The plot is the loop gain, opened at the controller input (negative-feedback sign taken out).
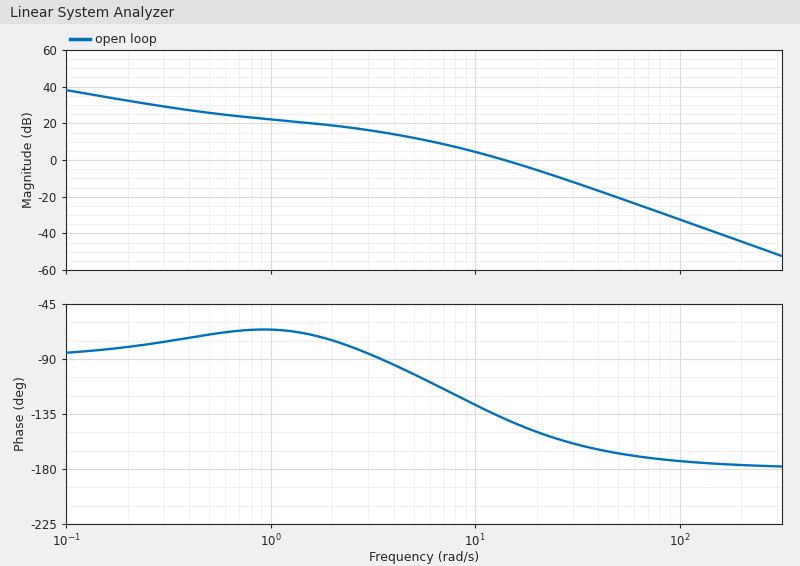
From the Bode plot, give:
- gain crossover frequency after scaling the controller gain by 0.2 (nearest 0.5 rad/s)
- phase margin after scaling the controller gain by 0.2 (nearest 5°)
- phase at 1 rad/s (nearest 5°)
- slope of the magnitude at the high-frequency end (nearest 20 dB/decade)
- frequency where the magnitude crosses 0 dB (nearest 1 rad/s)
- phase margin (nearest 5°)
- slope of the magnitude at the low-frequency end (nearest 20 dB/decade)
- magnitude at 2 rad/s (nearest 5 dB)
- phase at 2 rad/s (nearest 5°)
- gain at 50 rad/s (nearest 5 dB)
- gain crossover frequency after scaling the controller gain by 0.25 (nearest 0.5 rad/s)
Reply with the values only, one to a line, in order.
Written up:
4.0 rad/s
85°
-65°
-40 dB/decade
14 rad/s
40°
-20 dB/decade
20 dB
-75°
-20 dB
5.0 rad/s
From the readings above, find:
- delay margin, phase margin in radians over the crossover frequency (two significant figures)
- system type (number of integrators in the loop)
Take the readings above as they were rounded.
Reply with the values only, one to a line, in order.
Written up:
0.050 s
1
